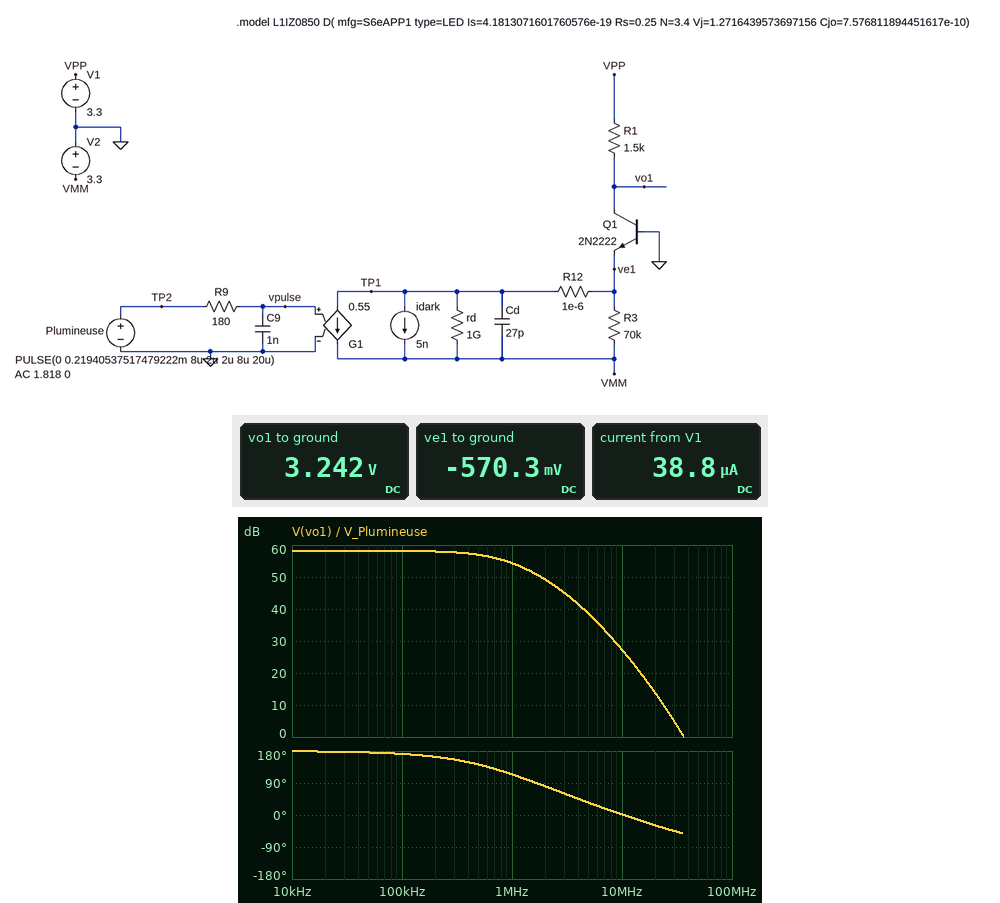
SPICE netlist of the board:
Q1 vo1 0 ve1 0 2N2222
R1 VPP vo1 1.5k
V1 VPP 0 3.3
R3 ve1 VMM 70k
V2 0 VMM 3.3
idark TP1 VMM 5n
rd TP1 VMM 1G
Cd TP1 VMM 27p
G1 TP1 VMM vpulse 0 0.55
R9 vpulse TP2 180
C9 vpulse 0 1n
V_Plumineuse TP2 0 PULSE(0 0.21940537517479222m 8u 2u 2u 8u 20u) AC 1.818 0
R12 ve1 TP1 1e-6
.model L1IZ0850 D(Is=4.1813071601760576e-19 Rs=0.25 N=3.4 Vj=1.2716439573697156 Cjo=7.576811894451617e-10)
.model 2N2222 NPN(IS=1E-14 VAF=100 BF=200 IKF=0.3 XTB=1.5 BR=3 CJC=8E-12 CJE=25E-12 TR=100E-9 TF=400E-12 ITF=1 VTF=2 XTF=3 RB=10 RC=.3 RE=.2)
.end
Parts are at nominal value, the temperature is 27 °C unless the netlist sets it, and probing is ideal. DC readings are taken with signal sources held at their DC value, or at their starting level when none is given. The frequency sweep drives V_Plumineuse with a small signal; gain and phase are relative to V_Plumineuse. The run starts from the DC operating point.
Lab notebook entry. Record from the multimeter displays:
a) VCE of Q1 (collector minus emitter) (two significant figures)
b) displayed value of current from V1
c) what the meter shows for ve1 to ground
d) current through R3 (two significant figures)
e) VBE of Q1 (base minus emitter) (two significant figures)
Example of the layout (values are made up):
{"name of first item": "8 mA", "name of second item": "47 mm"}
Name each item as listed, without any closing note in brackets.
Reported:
{"VCE of Q1 (collector minus emitter)": "3.8 V", "displayed value of current from V1": "38.8 µA", "what the meter shows for ve1 to ground": "-570.3 mV", "current through R3": "39 µA", "VBE of Q1 (base minus emitter)": "570 mV"}
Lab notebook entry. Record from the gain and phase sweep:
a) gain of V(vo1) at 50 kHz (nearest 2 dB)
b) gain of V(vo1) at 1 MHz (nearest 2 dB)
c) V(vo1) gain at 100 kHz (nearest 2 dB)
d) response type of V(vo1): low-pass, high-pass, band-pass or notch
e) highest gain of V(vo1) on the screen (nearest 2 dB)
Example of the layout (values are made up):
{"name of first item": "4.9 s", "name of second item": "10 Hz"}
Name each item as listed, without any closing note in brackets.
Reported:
{"gain of V(vo1) at 50 kHz": "58 dB", "gain of V(vo1) at 1 MHz": "54 dB", "V(vo1) gain at 100 kHz": "58 dB", "response type of V(vo1): low-pass, high-pass, band-pass or notch": "low-pass", "highest gain of V(vo1) on the screen": "58 dB"}
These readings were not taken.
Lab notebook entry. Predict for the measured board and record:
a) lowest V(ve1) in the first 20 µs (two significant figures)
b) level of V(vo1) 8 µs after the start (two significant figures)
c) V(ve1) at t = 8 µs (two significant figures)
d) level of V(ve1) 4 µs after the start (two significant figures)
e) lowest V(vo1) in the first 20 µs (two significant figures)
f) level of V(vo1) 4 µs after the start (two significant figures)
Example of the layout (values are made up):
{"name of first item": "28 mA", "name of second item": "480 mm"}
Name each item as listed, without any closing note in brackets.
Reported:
{"lowest V(ve1) in the first 20 µs": "-610 mV", "level of V(vo1) 8 µs after the start": "3.2 V", "V(ve1) at t = 8 µs": "-570 mV", "level of V(ve1) 4 µs after the start": "-570 mV", "lowest V(vo1) in the first 20 µs": "3.1 V", "level of V(vo1) 4 µs after the start": "3.2 V"}
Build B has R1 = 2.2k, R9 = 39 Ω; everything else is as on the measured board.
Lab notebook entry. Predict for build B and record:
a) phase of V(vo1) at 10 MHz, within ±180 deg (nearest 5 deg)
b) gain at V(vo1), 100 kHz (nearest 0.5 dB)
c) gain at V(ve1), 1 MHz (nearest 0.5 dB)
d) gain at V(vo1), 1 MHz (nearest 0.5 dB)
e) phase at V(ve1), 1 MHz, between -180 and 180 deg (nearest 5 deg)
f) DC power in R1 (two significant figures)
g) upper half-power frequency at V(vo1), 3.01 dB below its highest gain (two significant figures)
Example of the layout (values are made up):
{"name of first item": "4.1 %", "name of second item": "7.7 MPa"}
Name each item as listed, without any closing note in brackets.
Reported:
{"phase of V(vo1) at 10 MHz, within ±180 deg": "10 deg", "gain at V(vo1), 100 kHz": "61.5 dB", "gain at V(ve1), 1 MHz": "50.5 dB", "gain at V(vo1), 1 MHz": "61.0 dB", "phase at V(ve1), 1 MHz, between -180 and 180 deg": "150 deg", "DC power in R1": "3.3 µW", "upper half-power frequency at V(vo1), 3.01 dB below its highest gain": "2.5 MHz"}
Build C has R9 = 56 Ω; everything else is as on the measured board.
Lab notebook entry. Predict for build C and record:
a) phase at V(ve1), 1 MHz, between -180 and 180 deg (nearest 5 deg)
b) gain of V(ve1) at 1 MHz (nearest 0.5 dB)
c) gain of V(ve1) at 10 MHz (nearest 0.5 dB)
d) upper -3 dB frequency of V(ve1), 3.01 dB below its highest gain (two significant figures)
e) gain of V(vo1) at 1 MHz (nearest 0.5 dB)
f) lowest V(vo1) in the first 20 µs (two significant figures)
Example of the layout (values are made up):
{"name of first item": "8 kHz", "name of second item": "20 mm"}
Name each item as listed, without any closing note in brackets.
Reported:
{"phase at V(ve1), 1 MHz, between -180 and 180 deg": "145 deg", "gain of V(ve1) at 1 MHz": "50.5 dB", "gain of V(ve1) at 10 MHz": "31.0 dB", "upper -3 dB frequency of V(ve1), 3.01 dB below its highest gain": "2.1 MHz", "gain of V(vo1) at 1 MHz": "57.5 dB", "lowest V(vo1) in the first 20 µs": "3.1 V"}
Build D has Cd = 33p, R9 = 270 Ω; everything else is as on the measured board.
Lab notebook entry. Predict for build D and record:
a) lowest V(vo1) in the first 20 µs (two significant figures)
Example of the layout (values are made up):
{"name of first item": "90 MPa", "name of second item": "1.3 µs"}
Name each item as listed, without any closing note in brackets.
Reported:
{"lowest V(vo1) in the first 20 µs": "3.1 V"}
